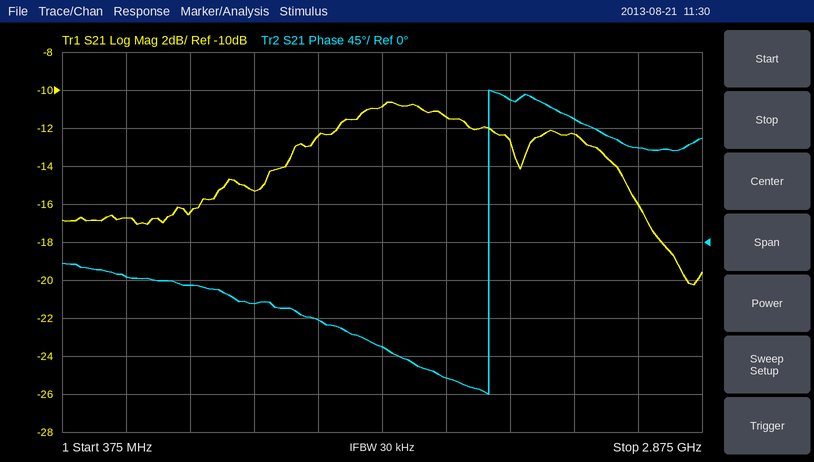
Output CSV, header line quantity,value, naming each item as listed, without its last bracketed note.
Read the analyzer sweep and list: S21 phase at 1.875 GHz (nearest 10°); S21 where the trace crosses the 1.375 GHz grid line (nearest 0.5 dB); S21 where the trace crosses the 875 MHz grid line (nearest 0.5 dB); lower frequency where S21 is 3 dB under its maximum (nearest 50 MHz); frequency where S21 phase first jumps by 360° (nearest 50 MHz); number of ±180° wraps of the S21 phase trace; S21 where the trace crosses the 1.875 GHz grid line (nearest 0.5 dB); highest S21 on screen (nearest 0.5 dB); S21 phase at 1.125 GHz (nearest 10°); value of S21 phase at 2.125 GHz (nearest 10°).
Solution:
quantity,value
S21 phase at 1.875 GHz,-160°
S21 where the trace crosses the 1.375 GHz grid line,-12.5 dB
S21 where the trace crosses the 875 MHz grid line,-16.5 dB
lower frequency where S21 is 3 dB under its maximum,1.25 GHz
frequency where S21 phase first jumps by 360°,2.05 GHz
number of ±180° wraps of the S21 phase trace,1
S21 where the trace crosses the 1.875 GHz grid line,-11.5 dB
highest S21 on screen,-10.5 dB
S21 phase at 1.125 GHz,-70°
value of S21 phase at 2.125 GHz,170°
